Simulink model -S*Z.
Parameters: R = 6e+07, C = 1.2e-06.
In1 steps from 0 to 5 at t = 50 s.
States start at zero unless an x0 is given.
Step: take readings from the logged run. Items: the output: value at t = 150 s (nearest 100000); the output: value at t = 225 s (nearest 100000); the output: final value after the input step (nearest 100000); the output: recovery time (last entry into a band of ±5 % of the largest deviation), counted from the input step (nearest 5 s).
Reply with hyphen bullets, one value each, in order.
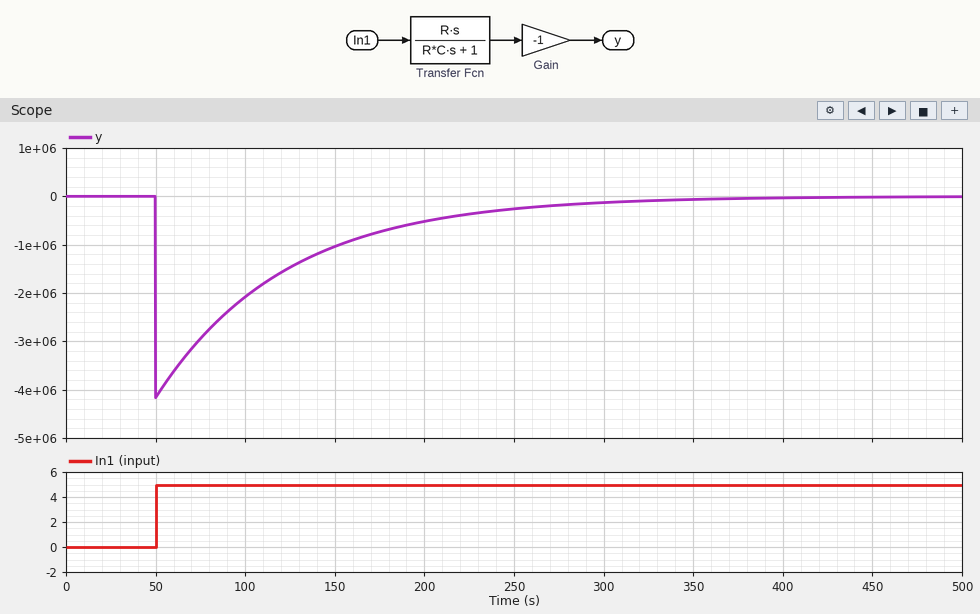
- -1000000
- -400000
- 0
- 215 s
